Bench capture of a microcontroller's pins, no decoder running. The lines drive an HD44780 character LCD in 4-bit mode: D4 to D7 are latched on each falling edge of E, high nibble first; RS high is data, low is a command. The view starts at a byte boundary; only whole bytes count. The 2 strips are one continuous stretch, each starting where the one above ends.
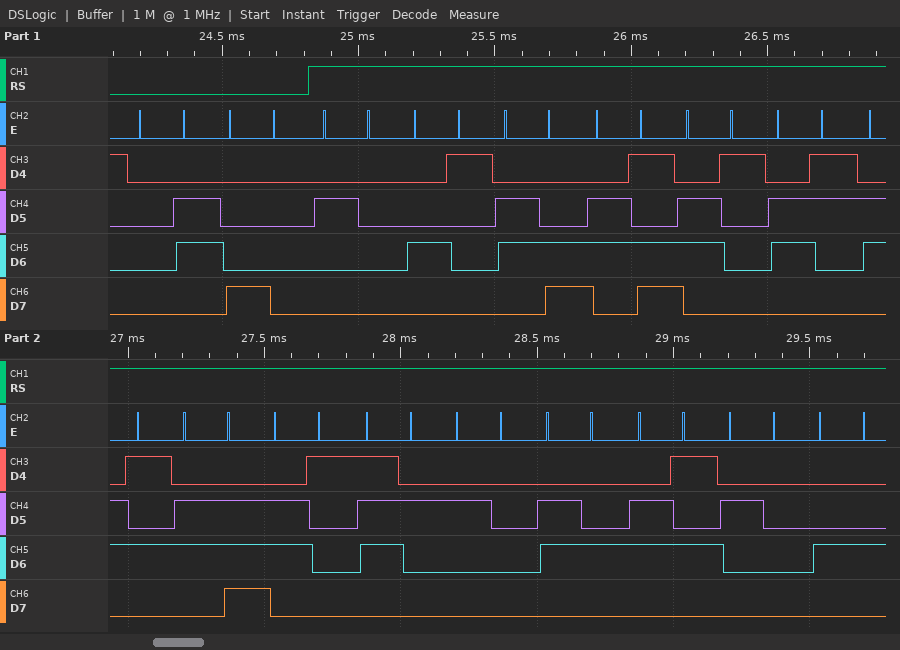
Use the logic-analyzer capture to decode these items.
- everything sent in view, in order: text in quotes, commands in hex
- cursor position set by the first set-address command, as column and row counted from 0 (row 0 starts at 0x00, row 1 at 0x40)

0x06 0x80 " Almacenar de D"
column 0, row 0
